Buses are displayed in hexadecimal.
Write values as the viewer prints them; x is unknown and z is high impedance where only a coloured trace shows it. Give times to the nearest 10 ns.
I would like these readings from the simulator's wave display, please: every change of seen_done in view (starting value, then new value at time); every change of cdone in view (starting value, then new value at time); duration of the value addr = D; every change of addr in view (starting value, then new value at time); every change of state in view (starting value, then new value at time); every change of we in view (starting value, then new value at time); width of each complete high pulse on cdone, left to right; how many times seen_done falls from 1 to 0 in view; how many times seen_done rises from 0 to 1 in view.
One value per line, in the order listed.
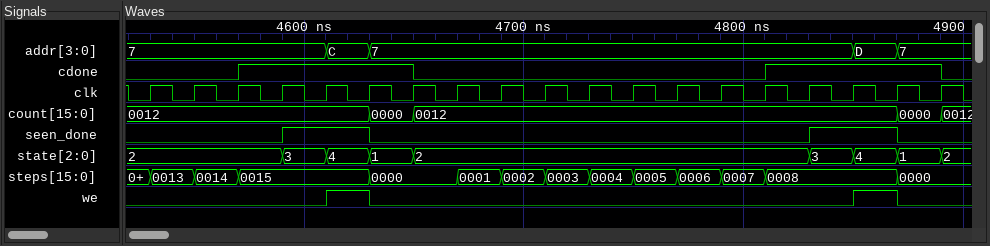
0, 1 at 4590 ns, 0 at 4630 ns, 1 at 4830 ns, 0 at 4870 ns
0, 1 at 4570 ns, 0 at 4650 ns, 1 at 4810 ns, 0 at 4890 ns
20 ns
7, C at 4610 ns, 7 at 4630 ns, D at 4850 ns, 7 at 4870 ns
2, 3 at 4590 ns, 4 at 4610 ns, 1 at 4630 ns, 2 at 4650 ns, 3 at 4830 ns, 4 at 4850 ns, 1 at 4870 ns, 2 at 4890 ns
0, 1 at 4610 ns, 0 at 4630 ns, 1 at 4850 ns, 0 at 4870 ns
80 ns, 80 ns
2
2
